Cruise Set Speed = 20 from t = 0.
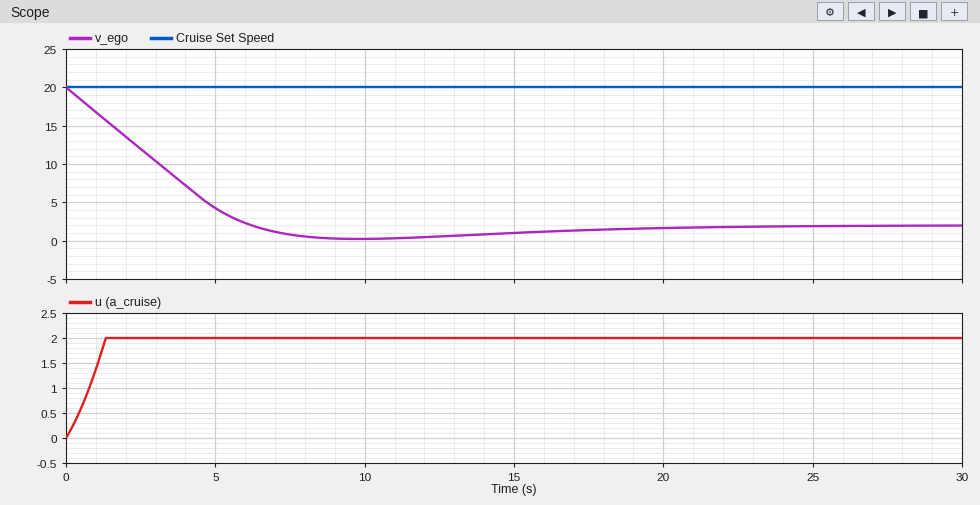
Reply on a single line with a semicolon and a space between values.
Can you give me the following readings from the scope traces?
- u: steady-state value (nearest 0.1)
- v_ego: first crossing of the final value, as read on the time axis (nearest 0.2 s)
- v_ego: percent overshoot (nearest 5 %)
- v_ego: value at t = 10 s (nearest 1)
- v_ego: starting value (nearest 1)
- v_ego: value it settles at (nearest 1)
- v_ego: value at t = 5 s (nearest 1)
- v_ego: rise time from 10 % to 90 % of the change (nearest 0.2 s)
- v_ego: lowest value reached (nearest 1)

2.0; 6.2 s; 10 %; 0; 20; 2; 4; 4.6 s; 0
